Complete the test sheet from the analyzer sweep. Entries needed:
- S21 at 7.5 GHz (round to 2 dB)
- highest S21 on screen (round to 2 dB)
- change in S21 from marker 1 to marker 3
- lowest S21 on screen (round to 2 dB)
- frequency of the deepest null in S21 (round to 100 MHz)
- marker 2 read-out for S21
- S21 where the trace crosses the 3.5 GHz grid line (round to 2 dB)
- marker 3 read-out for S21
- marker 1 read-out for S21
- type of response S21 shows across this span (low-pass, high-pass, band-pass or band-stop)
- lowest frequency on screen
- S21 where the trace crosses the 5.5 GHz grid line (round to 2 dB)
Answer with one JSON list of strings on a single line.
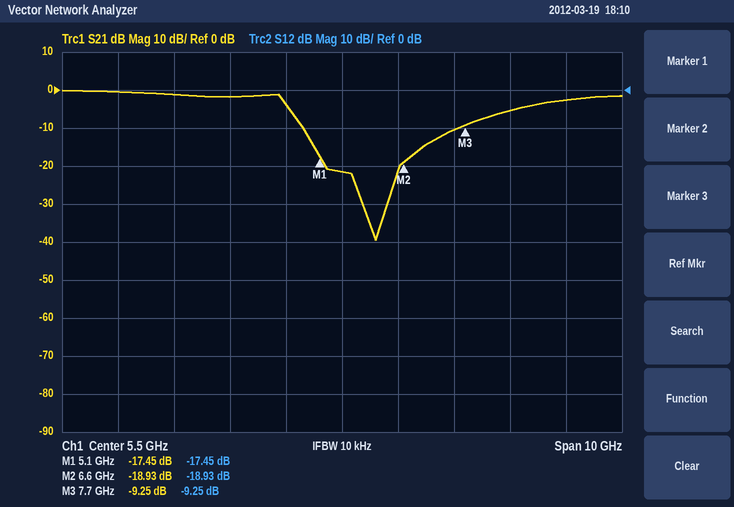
["-10 dB", "0 dB", "8.20 dB", "-40 dB", "6.1 GHz", "-18.93 dB", "-2 dB", "-9.25 dB", "-17.45 dB", "band-stop", "500 MHz", "-22 dB"]
